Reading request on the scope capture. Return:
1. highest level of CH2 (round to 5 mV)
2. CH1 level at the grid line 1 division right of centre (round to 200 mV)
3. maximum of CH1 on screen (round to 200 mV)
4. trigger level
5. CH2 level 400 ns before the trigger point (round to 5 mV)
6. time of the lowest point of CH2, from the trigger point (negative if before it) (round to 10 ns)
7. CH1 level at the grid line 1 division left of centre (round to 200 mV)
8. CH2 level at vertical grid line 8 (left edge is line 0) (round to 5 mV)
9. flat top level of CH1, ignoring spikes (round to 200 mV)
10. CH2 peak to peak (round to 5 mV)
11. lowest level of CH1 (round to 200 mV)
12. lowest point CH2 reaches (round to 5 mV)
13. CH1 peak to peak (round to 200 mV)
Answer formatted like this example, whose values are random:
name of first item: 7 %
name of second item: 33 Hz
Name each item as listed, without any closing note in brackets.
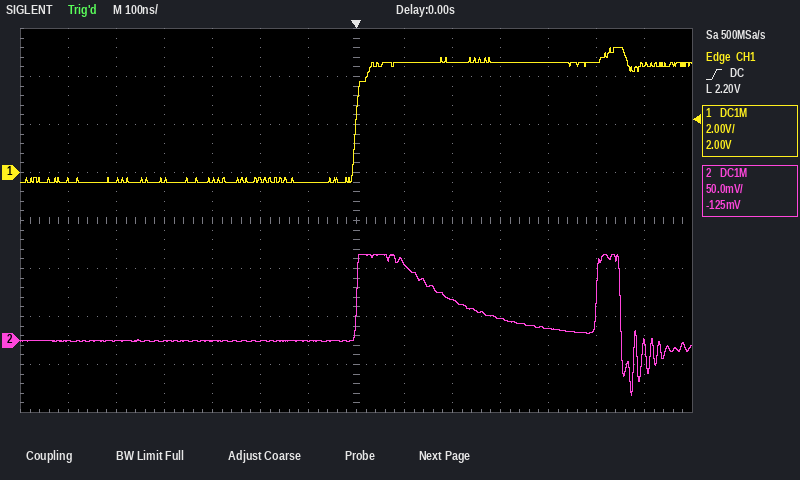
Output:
highest level of CH2: 90 mV
CH1 level at the grid line 1 division right of centre: 4.6 V
maximum of CH1 on screen: 5.2 V
trigger level: 2.20 V
CH2 level 400 ns before the trigger point: 0 mV
time of the lowest point of CH2, from the trigger point (negative if before it): +570 ns
CH1 level at the grid line 1 division left of centre: -400 mV
CH2 level at vertical grid line 8 (left edge is line 0): 80 mV
flat top level of CH1, ignoring spikes: 4.6 V
CH2 peak to peak: 145 mV
lowest level of CH1: -400 mV
lowest point CH2 reaches: -55 mV
CH1 peak to peak: 5.6 V
